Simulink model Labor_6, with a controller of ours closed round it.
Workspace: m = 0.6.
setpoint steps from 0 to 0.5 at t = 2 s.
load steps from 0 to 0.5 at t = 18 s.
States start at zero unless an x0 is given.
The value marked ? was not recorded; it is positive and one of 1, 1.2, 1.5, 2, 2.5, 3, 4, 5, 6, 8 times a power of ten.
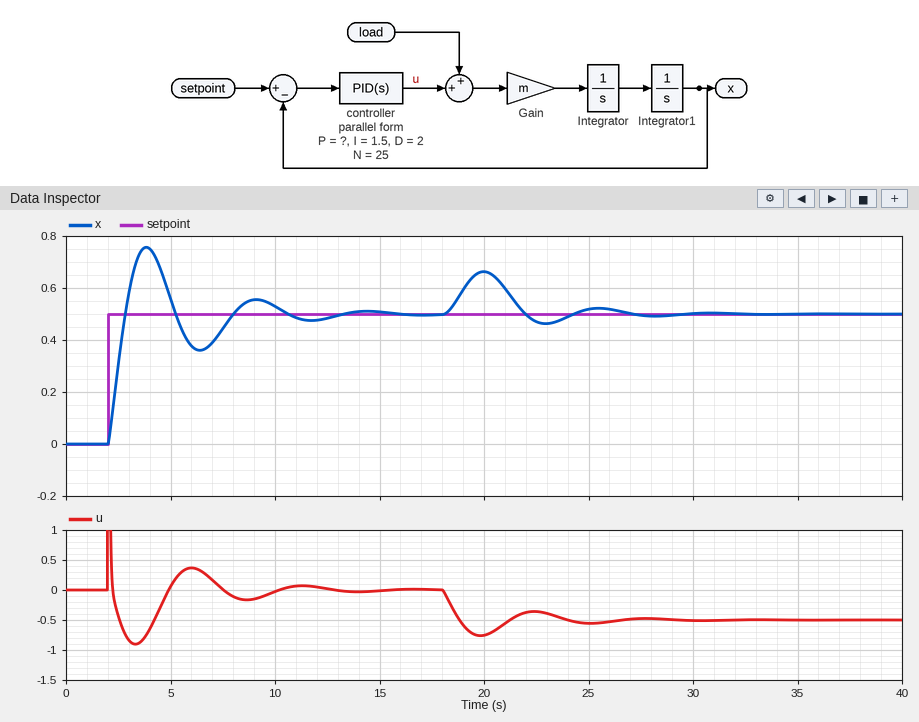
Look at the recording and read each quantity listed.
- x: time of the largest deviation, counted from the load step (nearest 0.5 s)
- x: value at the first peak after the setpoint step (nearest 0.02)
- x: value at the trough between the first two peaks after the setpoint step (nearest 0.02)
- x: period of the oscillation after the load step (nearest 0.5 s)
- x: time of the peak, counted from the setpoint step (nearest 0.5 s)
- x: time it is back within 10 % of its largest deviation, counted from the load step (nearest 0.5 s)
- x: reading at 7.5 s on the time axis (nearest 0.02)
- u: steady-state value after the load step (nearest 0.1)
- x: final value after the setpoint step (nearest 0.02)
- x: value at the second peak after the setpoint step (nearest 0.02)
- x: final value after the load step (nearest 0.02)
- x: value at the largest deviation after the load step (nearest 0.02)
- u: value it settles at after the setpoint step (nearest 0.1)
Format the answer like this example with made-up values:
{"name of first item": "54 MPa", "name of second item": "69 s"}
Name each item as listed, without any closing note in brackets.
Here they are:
{"x: time of the largest deviation, counted from the load step": "2.0 s", "x: value at the first peak after the setpoint step": "0.76", "x: value at the trough between the first two peaks after the setpoint step": "0.36", "x: period of the oscillation after the load step": "5.5 s", "x: time of the peak, counted from the setpoint step": "2.0 s", "x: time it is back within 10 % of its largest deviation, counted from the load step": "8.0 s", "x: reading at 7.5 s on the time axis": "0.44", "u: steady-state value after the load step": "-0.5", "x: final value after the setpoint step": "0.50", "x: value at the second peak after the setpoint step": "0.56", "x: final value after the load step": "0.50", "x: value at the largest deviation after the load step": "0.66", "u: value it settles at after the setpoint step": "0.0"}
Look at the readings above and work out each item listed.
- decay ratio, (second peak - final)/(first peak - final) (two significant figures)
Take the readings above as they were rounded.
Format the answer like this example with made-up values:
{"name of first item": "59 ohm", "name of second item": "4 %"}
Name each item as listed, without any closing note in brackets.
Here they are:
{"decay ratio, (second peak - final)/(first peak - final)": "0.23"}
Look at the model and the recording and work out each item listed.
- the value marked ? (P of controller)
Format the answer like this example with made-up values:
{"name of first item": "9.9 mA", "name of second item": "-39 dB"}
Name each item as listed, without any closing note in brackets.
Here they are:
{"the value marked ?": "3"}
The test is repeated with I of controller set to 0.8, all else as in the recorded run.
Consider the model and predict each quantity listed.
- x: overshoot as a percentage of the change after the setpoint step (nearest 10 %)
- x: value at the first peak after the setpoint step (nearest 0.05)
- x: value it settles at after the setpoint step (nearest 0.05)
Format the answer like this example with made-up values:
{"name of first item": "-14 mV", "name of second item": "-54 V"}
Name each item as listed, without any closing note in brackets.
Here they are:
{"x: overshoot as a percentage of the change after the setpoint step": "40 %", "x: value at the first peak after the setpoint step": "0.70", "x: value it settles at after the setpoint step": "0.50"}
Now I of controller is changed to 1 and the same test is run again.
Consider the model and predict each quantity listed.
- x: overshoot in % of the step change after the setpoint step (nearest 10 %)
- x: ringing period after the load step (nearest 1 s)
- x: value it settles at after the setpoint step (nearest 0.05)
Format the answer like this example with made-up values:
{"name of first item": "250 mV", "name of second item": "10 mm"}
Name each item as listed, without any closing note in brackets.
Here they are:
{"x: overshoot in % of the step change after the setpoint step": "50 %", "x: ringing period after the load step": "5 s", "x: value it settles at after the setpoint step": "0.50"}
